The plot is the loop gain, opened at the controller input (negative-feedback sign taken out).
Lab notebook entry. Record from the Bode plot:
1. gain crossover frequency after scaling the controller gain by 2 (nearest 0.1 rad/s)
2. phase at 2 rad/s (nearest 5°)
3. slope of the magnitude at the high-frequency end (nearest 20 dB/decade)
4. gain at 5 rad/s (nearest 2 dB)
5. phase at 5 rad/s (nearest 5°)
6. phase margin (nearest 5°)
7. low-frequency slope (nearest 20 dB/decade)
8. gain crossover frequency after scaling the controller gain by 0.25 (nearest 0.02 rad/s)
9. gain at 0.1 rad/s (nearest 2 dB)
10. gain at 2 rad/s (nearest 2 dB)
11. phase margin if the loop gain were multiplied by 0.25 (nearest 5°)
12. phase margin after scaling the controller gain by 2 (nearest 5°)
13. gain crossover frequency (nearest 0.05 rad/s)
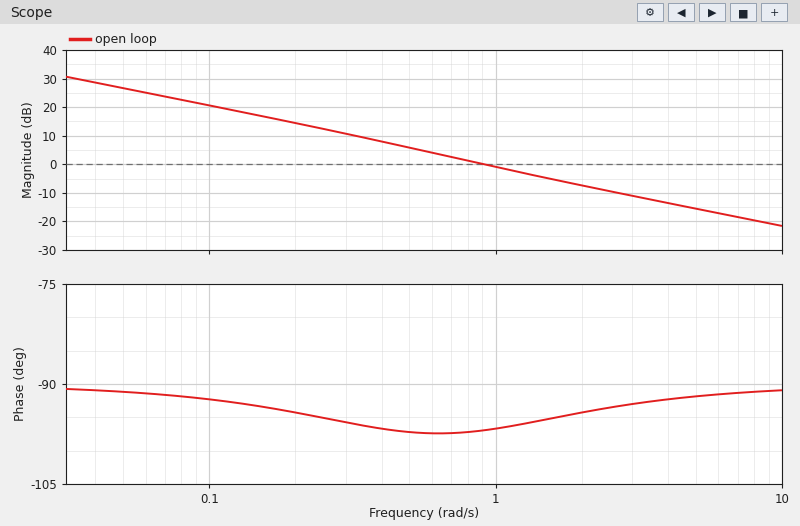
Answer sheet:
1.7 rad/s
-95°
-20 dB/decade
-16 dB
-90°
85°
-20 dB/decade
0.26 rad/s
20 dB
-8 dB
85°
85°
0.90 rad/s
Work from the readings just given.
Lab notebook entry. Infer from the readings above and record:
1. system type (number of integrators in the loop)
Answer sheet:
1
